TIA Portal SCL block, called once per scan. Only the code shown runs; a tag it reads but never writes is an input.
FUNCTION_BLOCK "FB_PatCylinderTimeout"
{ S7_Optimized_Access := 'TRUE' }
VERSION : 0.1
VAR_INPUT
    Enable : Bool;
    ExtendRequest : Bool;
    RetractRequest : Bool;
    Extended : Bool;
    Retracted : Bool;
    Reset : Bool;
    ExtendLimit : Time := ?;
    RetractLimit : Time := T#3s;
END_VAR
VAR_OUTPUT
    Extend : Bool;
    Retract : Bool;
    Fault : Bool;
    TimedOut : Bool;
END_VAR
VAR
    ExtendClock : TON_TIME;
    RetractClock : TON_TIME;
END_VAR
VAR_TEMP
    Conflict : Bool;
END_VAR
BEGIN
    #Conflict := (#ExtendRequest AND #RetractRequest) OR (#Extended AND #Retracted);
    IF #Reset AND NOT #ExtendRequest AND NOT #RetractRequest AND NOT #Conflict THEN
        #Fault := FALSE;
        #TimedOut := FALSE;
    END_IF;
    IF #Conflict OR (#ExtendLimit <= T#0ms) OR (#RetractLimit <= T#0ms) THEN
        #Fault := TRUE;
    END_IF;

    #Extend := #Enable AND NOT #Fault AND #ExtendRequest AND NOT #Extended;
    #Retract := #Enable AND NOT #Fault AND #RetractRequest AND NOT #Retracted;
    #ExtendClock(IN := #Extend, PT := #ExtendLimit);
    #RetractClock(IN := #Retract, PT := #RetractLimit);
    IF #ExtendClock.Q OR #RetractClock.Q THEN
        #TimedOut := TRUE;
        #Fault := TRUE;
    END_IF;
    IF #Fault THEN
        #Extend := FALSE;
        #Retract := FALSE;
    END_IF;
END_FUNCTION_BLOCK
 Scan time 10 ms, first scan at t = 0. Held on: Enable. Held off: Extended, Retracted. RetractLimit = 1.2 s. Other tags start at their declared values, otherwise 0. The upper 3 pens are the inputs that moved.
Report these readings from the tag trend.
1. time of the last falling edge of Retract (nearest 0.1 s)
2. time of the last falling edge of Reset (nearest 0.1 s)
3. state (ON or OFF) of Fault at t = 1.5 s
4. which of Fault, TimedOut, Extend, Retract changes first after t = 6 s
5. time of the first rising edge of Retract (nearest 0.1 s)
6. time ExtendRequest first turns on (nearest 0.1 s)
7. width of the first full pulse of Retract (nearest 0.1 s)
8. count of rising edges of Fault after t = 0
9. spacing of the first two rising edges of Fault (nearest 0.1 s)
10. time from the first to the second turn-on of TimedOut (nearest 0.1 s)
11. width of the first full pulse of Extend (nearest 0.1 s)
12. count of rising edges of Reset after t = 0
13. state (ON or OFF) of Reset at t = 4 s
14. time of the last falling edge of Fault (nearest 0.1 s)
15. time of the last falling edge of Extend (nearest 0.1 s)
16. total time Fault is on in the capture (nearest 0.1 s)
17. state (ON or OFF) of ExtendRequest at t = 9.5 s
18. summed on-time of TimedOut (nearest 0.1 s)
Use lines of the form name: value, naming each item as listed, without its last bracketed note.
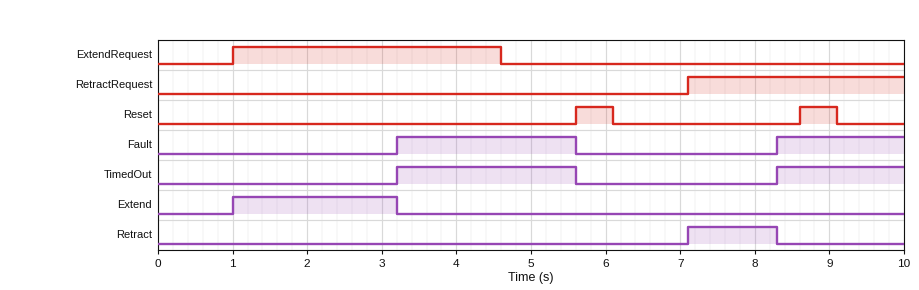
time of the last falling edge of Retract: 8.3 s
time of the last falling edge of Reset: 9.1 s
state (ON or OFF) of Fault at t = 1.5 s: OFF
which of Fault, TimedOut, Extend, Retract changes first after t = 6 s: Retract
time of the first rising edge of Retract: 7.1 s
time ExtendRequest first turns on: 1.0 s
width of the first full pulse of Retract: 1.2 s
count of rising edges of Fault after t = 0: 2
spacing of the first two rising edges of Fault: 5.1 s
time from the first to the second turn-on of TimedOut: 5.1 s
width of the first full pulse of Extend: 2.2 s
count of rising edges of Reset after t = 0: 2
state (ON or OFF) of Reset at t = 4 s: OFF
time of the last falling edge of Fault: 5.6 s
time of the last falling edge of Extend: 3.2 s
total time Fault is on in the capture: 4.1 s
state (ON or OFF) of ExtendRequest at t = 9.5 s: OFF
summed on-time of TimedOut: 4.1 s
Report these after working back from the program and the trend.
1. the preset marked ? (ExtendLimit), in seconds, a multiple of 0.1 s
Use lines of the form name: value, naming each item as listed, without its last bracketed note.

the preset marked ? (ExtendLimit), in seconds, a multiple of 0.1 s: 2.2 s
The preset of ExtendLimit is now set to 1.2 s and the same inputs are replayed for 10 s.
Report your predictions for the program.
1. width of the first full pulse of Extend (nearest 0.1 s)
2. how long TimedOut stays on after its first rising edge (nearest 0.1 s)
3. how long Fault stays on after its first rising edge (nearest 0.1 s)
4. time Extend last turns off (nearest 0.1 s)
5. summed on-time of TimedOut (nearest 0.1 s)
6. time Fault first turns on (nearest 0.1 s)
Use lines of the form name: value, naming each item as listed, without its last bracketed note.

width of the first full pulse of Extend: 1.2 s
how long TimedOut stays on after its first rising edge: 3.4 s
how long Fault stays on after its first rising edge: 3.4 s
time Extend last turns off: 2.2 s
summed on-time of TimedOut: 5.1 s
time Fault first turns on: 2.2 s
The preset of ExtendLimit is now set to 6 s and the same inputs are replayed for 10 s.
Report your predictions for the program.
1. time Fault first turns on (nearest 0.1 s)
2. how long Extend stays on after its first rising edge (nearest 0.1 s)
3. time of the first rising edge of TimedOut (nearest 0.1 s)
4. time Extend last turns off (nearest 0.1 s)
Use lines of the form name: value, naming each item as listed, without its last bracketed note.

time Fault first turns on: 8.3 s
how long Extend stays on after its first rising edge: 3.6 s
time of the first rising edge of TimedOut: 8.3 s
time Extend last turns off: 4.6 s
